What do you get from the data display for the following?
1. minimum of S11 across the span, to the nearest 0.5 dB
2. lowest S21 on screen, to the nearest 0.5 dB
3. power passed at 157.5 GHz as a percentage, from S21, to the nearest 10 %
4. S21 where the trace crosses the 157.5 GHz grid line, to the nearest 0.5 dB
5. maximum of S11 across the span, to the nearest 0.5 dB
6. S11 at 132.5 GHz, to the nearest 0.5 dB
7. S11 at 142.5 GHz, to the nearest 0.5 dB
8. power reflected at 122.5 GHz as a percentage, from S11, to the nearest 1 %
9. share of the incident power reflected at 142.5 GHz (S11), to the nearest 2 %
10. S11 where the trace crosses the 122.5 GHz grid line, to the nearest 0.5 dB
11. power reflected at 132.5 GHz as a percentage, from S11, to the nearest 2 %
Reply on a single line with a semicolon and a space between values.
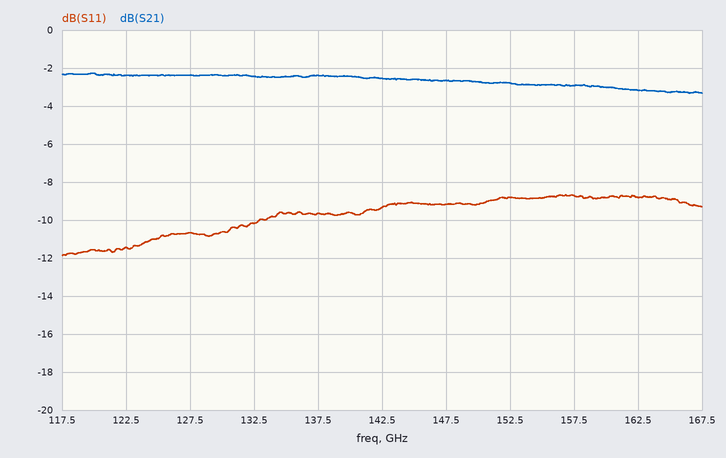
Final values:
-12.0 dB; -3.5 dB; 50 %; -3.0 dB; -8.5 dB; -10.0 dB; -9.5 dB; 7 %; 12 %; -11.5 dB; 10 %
